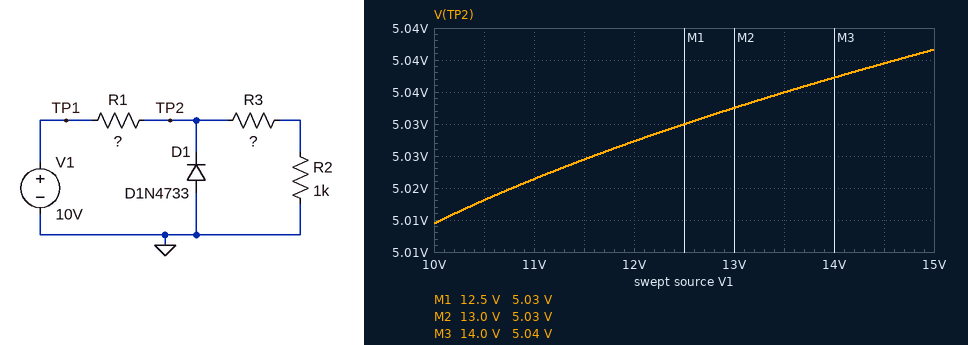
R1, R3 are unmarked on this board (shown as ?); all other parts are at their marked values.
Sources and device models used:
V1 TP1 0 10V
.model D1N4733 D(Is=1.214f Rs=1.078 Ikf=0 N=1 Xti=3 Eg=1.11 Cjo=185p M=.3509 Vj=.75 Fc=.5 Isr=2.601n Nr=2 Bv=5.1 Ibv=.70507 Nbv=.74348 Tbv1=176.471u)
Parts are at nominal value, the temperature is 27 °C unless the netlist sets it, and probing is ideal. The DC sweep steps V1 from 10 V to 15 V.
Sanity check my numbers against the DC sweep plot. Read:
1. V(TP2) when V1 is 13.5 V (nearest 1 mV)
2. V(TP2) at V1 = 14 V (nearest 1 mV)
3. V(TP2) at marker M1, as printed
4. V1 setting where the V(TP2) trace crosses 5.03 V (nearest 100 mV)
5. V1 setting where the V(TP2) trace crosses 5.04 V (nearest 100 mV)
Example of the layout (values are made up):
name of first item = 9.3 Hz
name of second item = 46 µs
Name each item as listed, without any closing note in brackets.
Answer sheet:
V(TP2) when V1 is 13.5 V = 5.035 V
V(TP2) at V1 = 14 V = 5.037 V
V(TP2) at marker M1, as printed = 5.03 V
V1 setting where the V(TP2) trace crosses 5.03 V = 12.5 V
V1 setting where the V(TP2) trace crosses 5.04 V = 13.5 V
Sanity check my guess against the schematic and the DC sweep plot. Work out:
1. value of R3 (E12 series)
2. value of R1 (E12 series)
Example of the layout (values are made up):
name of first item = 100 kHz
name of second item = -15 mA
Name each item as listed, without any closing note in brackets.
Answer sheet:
value of R3 = 680 Ω
value of R1 = 560 Ω
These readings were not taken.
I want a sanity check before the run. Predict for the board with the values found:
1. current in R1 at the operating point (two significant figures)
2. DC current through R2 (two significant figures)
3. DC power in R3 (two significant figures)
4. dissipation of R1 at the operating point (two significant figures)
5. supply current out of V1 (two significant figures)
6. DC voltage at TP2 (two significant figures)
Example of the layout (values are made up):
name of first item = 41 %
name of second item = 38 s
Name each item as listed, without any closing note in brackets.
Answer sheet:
current in R1 at the operating point = 8.9 mA
DC current through R2 = 3.0 mA
DC power in R3 = 6.1 mW
dissipation of R1 at the operating point = 44 mW
supply current out of V1 = 8.9 mA
DC voltage at TP2 = 5.0 V
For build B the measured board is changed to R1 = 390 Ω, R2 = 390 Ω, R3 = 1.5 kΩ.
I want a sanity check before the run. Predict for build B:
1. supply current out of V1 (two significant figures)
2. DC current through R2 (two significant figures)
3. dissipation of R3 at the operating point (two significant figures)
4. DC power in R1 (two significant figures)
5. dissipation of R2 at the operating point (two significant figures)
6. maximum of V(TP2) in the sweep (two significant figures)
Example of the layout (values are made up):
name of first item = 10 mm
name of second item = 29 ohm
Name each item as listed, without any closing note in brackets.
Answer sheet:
supply current out of V1 = 13 mA
DC current through R2 = 2.7 mA
dissipation of R3 at the operating point = 11 mW
DC power in R1 = 63 mW
dissipation of R2 at the operating point = 2.8 mW
maximum of V(TP2) in the sweep = 5.1 V
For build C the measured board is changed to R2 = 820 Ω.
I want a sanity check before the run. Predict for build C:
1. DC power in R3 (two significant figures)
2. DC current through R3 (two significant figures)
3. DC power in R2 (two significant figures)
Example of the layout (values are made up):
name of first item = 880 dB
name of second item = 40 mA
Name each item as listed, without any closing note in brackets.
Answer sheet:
DC power in R3 = 7.6 mW
DC current through R3 = 3.3 mA
DC power in R2 = 9.2 mW
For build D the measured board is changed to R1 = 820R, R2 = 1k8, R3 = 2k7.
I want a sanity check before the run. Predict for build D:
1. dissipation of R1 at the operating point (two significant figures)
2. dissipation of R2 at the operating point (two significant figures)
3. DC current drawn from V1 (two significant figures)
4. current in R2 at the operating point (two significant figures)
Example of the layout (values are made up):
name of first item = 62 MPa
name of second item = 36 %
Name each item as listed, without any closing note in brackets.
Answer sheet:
dissipation of R1 at the operating point = 30 mW
dissipation of R2 at the operating point = 2.2 mW
DC current drawn from V1 = 6.1 mA
current in R2 at the operating point = 1.1 mA
